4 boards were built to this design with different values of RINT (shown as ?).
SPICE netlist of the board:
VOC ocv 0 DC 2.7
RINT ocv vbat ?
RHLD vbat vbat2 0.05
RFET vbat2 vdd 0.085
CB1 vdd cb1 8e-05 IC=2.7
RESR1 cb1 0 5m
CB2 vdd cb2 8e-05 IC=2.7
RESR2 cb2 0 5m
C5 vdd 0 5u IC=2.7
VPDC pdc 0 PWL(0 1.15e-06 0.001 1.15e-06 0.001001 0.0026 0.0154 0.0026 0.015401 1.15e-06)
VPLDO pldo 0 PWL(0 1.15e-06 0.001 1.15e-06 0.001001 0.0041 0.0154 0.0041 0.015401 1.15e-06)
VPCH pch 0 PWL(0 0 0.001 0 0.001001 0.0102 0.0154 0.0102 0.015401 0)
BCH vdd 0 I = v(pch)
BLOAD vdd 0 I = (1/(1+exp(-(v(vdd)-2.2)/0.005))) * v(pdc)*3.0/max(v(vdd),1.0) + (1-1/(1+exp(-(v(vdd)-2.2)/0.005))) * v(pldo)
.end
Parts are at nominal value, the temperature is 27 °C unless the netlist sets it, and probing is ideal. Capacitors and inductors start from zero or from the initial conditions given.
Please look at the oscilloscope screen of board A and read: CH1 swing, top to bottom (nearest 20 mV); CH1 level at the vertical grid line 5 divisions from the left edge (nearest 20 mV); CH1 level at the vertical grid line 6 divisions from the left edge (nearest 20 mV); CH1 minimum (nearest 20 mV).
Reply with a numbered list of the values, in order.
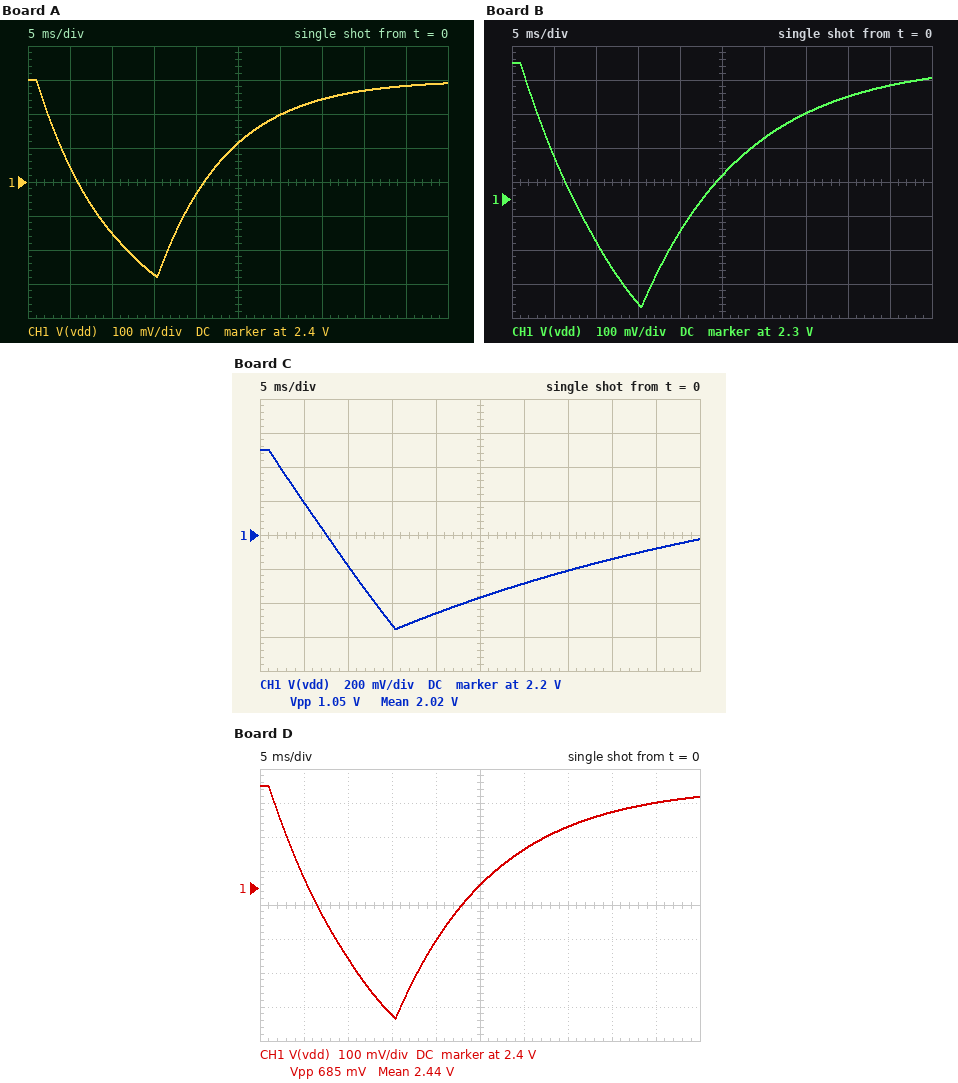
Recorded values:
1. 580 mV
2. 2.52 V
3. 2.60 V
4. 2.12 V
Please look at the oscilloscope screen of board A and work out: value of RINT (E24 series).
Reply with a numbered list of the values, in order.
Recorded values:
1. 51 Ω
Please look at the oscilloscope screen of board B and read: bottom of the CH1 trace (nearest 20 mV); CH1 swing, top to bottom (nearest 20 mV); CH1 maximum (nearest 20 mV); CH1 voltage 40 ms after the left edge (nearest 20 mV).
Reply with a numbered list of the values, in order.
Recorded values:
1. 1.98 V
2. 720 mV
3. 2.70 V
4. 2.60 V
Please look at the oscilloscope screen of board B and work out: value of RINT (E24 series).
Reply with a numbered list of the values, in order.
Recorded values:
1. 75 Ω
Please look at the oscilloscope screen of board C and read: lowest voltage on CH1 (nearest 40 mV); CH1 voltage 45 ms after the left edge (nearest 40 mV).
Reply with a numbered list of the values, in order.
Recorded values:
1. 1.64 V
2. 2.12 V
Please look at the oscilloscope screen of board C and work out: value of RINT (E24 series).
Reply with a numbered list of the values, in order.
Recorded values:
1. 300 Ω
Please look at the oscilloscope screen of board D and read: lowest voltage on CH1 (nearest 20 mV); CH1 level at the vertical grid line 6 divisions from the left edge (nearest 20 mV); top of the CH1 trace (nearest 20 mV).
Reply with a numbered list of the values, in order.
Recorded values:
1. 2.02 V
2. 2.52 V
3. 2.70 V
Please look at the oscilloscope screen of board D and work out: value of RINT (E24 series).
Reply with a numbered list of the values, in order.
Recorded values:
1. 68 Ω
